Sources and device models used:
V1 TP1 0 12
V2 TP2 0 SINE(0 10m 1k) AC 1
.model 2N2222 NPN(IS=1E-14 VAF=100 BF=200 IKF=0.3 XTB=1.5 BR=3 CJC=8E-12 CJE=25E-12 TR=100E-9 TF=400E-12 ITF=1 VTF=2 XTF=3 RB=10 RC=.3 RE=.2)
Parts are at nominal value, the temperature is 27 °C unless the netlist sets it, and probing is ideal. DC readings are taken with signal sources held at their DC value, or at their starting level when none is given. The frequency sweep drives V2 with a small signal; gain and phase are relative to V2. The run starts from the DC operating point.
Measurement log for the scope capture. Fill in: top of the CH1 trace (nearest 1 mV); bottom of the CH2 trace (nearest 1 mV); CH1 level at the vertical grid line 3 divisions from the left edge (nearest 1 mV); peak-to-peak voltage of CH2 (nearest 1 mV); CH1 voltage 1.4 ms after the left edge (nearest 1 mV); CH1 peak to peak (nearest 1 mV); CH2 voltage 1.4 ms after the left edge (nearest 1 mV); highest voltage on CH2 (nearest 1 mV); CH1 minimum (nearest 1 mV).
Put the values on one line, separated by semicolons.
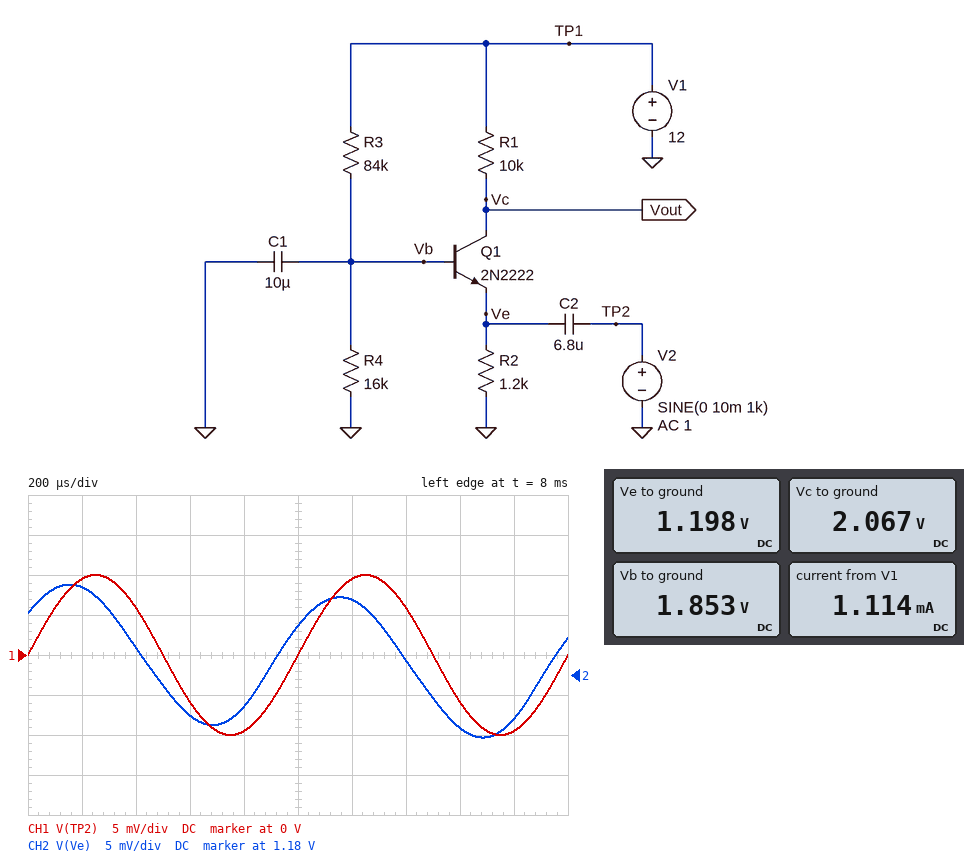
10 mV; 1.172 V; -6 mV; 19 mV; 6 mV; 20 mV; 1.182 V; 1.191 V; -10 mV
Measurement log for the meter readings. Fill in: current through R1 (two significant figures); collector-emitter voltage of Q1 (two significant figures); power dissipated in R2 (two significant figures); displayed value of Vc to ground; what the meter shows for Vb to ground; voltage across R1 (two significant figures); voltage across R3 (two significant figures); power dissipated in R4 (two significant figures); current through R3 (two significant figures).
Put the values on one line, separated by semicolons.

990 µA; 870 mV; 1.2 mW; 2.067 V; 1.853 V; 9.9 V; 10 V; 210 µW; 120 µA
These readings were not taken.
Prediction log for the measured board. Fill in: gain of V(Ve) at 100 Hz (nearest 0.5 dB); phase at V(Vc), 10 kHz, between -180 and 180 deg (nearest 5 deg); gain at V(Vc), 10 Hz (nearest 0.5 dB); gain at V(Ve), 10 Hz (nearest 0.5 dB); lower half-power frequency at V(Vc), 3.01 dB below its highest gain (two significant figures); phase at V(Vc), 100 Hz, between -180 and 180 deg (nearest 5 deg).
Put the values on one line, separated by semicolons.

-18.5 dB; 5 deg; 12.5 dB; -38.0 dB; 830 Hz; 85 deg
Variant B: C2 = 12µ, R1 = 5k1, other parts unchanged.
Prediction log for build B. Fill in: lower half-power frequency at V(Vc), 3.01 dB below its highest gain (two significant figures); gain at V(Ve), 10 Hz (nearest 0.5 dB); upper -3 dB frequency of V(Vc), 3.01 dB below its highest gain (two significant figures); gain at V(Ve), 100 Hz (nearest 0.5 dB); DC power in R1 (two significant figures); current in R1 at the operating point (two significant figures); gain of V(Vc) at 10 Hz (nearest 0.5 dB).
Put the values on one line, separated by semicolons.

500 Hz; -33.5 dB; 5.8 MHz; -14.0 dB; 5.1 mW; 1.0 mA; 11.5 dB
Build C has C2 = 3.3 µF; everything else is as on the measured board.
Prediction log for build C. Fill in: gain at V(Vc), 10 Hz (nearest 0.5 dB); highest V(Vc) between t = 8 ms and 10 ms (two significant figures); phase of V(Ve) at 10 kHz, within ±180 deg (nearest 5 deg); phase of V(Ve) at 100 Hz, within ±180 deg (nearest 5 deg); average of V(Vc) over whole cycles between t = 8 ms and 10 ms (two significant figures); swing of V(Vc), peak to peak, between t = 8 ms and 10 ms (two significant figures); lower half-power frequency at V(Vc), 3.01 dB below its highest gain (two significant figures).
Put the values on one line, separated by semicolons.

6.0 dB; 3.8 V; 10 deg; 85 deg; 2.3 V; 2.6 V; 1.7 kHz
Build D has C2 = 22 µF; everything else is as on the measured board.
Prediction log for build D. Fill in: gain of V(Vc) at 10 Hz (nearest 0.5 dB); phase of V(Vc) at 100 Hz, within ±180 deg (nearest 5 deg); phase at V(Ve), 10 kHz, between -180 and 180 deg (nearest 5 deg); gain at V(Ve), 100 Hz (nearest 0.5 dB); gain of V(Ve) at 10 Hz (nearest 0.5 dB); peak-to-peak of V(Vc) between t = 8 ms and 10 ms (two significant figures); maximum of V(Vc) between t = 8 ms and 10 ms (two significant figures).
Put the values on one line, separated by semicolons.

22.5 dB; 70 deg; 0 deg; -9.0 dB; -27.5 dB; 3.9 V; 5.1 V
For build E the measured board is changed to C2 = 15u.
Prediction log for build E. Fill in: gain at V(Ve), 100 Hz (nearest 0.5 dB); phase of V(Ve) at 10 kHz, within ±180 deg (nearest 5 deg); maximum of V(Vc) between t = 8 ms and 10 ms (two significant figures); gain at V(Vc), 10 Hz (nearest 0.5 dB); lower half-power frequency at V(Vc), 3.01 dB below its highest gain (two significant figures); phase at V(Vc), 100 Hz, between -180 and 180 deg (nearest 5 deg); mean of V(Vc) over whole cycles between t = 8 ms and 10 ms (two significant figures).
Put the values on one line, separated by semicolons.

-12.0 dB; 0 deg; 5.0 V; 19.0 dB; 380 Hz; 75 deg; 2.7 V
